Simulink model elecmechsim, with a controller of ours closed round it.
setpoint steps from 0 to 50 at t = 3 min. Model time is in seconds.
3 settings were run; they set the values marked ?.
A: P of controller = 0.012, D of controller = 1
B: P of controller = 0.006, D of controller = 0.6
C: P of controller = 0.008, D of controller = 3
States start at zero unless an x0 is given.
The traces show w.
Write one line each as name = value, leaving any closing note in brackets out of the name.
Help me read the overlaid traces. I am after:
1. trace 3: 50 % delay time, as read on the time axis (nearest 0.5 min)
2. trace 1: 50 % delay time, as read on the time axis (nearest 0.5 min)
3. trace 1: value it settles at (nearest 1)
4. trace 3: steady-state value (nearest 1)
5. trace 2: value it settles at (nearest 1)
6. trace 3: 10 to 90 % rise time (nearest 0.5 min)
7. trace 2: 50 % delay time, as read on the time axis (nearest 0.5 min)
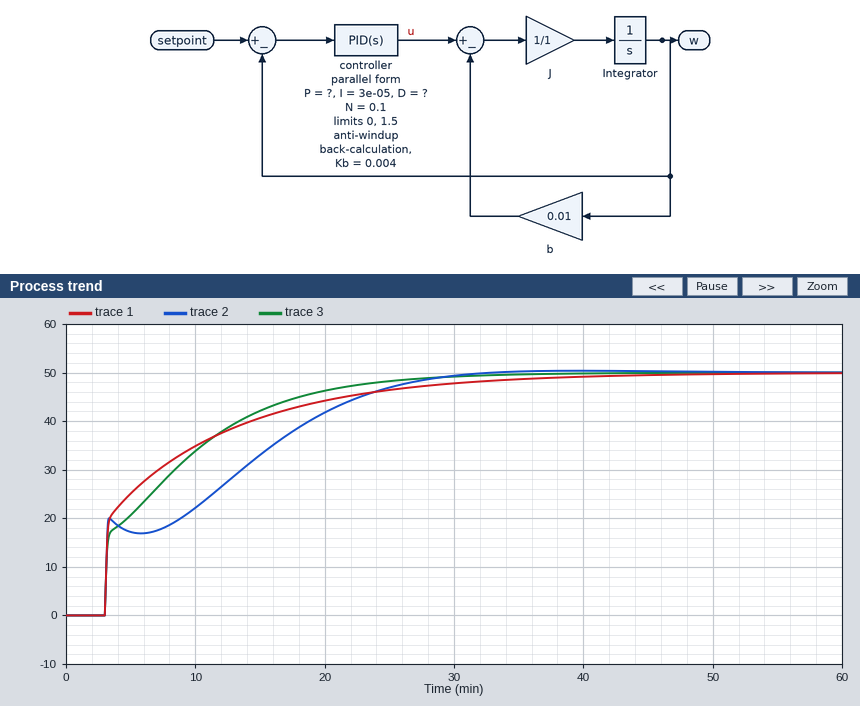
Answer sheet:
trace 3: 50 % delay time, as read on the time axis = 6.5 min
trace 1: 50 % delay time, as read on the time axis = 5.0 min
trace 1: value it settles at = 50
trace 3: steady-state value = 50
trace 2: value it settles at = 50
trace 3: 10 to 90 % rise time = 15.0 min
trace 2: 50 % delay time, as read on the time axis = 11.5 min
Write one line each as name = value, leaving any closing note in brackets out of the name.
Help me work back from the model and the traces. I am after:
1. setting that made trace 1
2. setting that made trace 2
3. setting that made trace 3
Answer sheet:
setting that made trace 1 = A
setting that made trace 2 = C
setting that made trace 3 = B
